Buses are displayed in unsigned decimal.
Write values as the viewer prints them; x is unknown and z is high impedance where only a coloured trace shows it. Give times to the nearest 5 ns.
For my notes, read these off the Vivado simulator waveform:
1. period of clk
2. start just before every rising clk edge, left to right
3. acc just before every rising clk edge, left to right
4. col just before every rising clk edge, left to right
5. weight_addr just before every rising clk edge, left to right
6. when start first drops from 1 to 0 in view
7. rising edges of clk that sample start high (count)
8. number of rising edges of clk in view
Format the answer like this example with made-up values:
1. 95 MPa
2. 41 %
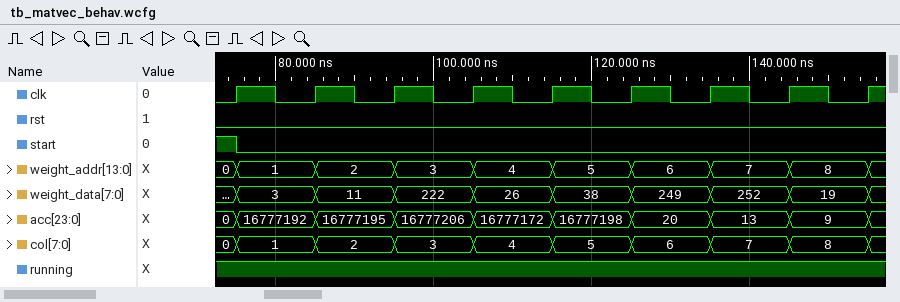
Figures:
1. 10 ns
2. 1 0 0 0 0 0 0 0 0
3. 0, 16777192, 16777195, 16777206, 16777172, 16777198, 20, 13, 9
4. 0, 1, 2, 3, 4, 5, 6, 7, 8
5. 0, 1, 2, 3, 4, 5, 6, 7, 8
6. 75 ns
7. 1
8. 9
